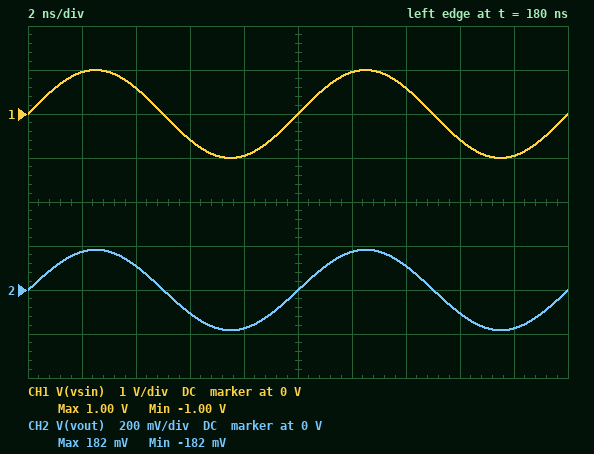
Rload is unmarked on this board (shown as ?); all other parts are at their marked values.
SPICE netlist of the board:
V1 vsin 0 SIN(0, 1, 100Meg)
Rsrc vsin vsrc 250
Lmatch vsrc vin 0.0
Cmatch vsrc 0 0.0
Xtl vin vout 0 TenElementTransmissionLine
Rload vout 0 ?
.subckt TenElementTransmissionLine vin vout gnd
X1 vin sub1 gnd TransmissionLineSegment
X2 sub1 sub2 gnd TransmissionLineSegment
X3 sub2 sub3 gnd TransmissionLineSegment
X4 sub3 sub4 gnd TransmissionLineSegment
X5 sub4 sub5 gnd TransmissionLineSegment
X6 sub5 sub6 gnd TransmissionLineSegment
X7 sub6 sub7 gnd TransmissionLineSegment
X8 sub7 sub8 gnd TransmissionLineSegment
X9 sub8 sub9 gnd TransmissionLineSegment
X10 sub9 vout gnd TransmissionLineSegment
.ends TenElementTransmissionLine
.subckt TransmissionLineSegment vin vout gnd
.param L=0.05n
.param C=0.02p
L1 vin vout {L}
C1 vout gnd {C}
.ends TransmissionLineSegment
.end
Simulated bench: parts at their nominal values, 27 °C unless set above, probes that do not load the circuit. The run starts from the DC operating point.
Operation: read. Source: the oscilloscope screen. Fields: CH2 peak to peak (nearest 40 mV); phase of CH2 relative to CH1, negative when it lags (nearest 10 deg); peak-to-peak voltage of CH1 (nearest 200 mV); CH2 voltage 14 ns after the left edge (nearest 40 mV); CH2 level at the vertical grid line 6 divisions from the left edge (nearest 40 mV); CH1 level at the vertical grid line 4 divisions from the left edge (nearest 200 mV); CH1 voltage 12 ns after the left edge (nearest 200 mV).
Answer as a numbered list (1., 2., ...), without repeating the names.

1. 360 mV
2. 0 deg
3. 2.0 V
4. 120 mV
5. 160 mV
6. -1.0 V
7. 1.0 V
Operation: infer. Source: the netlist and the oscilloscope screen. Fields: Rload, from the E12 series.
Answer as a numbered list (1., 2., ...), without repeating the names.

1. 56 Ω
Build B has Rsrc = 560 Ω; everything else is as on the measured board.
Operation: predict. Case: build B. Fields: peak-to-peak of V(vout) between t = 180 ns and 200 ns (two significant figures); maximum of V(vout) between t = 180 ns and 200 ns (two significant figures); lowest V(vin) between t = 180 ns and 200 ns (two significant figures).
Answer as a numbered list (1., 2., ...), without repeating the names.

1. 180 mV
2. 91 mV
3. -91 mV
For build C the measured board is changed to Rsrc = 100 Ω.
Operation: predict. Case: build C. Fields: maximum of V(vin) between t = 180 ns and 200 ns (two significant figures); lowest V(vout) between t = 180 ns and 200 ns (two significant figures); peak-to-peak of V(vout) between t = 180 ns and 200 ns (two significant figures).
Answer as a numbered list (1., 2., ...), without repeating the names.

1. 360 mV
2. -360 mV
3. 720 mV
